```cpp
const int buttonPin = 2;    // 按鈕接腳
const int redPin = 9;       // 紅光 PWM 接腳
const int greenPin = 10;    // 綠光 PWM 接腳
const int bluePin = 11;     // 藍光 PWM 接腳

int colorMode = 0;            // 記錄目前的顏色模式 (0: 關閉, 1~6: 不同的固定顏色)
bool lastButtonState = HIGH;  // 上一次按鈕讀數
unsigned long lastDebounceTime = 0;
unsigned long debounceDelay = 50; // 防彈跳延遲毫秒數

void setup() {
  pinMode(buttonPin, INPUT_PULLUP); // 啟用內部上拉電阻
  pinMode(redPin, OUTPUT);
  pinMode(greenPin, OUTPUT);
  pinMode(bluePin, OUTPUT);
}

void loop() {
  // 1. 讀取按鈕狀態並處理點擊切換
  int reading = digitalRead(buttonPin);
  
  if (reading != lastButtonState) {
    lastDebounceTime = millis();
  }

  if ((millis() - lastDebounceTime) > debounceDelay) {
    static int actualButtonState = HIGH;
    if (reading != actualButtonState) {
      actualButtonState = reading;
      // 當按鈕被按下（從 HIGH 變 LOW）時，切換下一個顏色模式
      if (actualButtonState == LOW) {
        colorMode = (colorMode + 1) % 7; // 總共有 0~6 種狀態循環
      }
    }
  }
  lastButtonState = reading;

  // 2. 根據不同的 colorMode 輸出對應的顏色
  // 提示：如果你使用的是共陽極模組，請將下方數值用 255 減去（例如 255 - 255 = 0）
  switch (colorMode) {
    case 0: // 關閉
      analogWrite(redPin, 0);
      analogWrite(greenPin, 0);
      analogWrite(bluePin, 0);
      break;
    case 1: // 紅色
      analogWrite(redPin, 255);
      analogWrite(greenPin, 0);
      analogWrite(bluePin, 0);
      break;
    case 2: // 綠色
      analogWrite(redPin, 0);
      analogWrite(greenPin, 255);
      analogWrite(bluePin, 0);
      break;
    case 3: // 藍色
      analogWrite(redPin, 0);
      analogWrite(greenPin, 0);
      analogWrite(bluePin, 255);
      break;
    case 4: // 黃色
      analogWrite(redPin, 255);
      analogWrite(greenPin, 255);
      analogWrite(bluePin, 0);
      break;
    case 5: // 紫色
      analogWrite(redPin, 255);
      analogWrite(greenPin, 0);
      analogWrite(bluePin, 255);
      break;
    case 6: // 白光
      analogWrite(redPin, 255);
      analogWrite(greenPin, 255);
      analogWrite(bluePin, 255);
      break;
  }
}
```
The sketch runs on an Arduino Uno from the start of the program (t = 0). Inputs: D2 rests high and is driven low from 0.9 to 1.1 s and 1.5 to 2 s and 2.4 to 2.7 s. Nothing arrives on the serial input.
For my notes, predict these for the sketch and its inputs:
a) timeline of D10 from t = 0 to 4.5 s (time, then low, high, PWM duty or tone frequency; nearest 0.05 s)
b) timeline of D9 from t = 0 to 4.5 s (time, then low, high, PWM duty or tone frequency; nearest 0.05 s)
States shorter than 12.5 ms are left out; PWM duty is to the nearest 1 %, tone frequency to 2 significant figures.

0 s low; 1.55 s high; 2.45 s low
0 s low; 0.95 s high; 1.55 s low
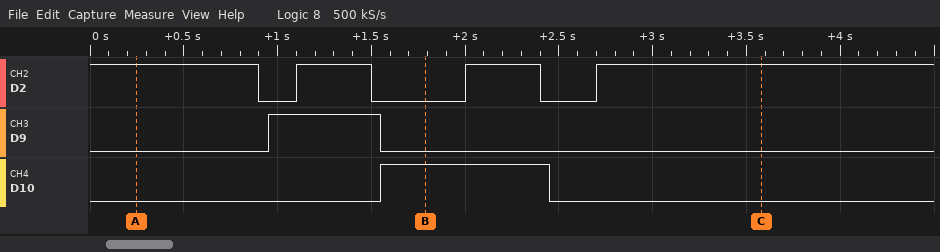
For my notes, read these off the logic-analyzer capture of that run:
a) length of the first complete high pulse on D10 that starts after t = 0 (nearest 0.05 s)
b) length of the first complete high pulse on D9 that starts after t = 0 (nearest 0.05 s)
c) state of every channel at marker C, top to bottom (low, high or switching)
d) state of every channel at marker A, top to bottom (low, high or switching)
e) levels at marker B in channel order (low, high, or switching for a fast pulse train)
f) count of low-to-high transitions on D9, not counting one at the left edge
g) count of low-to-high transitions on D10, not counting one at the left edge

0.90 s
0.60 s
D2 high, D9 low, D10 low
D2 high, D9 low, D10 low
D2 low, D9 low, D10 high
1
1
